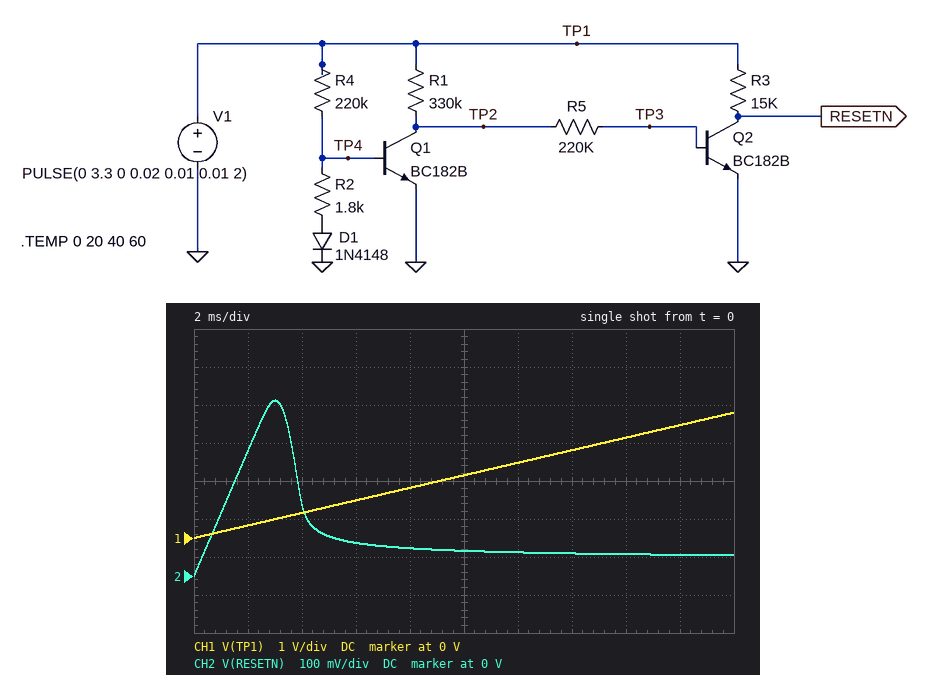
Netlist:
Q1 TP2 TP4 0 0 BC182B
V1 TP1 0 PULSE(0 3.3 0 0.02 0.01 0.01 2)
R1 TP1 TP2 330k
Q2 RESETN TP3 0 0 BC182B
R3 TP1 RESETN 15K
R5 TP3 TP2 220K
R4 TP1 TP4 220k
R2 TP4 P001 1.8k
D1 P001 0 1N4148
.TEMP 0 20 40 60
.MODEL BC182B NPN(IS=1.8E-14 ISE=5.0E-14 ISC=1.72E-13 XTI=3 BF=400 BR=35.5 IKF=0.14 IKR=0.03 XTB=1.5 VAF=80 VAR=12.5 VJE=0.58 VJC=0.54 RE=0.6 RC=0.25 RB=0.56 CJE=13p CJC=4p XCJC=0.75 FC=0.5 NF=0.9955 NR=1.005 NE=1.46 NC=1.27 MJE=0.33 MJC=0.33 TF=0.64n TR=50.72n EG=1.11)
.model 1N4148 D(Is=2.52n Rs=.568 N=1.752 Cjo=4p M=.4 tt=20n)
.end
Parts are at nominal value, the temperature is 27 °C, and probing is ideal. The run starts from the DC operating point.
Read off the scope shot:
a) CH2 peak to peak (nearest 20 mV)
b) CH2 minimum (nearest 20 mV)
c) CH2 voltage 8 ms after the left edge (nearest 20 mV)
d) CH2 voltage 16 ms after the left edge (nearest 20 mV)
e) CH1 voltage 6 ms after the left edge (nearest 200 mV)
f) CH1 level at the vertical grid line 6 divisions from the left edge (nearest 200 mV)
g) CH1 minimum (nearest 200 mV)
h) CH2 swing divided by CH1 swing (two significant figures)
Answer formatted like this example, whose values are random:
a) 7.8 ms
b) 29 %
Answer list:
a) 460 mV
b) 0 V
c) 80 mV
d) 60 mV
e) 1.0 V
f) 2.0 V
g) 0 V
h) 0.14
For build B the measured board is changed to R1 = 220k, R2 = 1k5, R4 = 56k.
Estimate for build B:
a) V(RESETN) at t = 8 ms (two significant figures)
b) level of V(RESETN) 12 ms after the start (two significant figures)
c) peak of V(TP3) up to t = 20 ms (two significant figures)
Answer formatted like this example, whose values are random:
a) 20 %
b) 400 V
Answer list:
a) 66 mV
b) 60 mV
c) 600 mV
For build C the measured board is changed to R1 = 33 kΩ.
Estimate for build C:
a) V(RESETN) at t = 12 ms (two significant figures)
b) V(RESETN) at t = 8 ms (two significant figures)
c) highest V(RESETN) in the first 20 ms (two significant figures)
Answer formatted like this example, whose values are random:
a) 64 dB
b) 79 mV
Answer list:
a) 37 mV
b) 45 mV
c) 450 mV
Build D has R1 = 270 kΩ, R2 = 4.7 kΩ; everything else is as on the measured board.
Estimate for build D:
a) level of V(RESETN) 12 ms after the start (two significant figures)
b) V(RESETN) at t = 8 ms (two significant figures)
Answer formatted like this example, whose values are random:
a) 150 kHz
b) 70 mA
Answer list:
a) 58 mV
b) 68 mV
